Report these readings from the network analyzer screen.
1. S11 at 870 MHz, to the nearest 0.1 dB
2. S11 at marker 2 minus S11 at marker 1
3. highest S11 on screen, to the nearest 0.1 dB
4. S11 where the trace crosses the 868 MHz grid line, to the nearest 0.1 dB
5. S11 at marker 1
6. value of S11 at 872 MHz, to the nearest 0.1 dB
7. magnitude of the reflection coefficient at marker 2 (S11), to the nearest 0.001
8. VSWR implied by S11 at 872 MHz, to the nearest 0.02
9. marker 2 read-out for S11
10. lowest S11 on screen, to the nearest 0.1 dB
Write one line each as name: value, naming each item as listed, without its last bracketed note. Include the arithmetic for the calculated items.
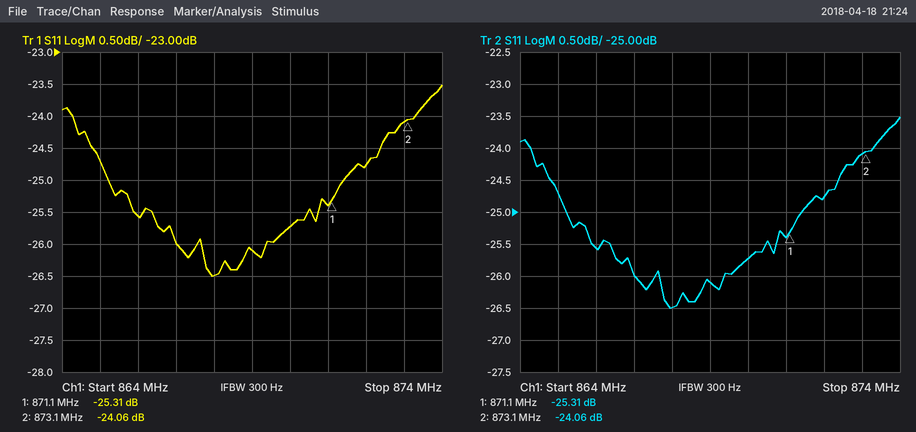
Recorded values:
S11 at 870 MHz, to the nearest 0.1 dB: -25.7 dB
S11 at marker 2 minus S11 at marker 1: -24.06 − (-25.31) = 1.25 dB
highest S11 on screen, to the nearest 0.1 dB: -23.5 dB
S11 where the trace crosses the 868 MHz grid line, to the nearest 0.1 dB: -26.5 dB
S11 at marker 1: -25.31 dB
value of S11 at 872 MHz, to the nearest 0.1 dB: -24.8 dB
magnitude of the reflection coefficient at marker 2 (S11), to the nearest 0.001: 10^(-24.06/20) ≈ 0.063
VSWR implied by S11 at 872 MHz, to the nearest 0.02: |Γ| = 10^(-24.8/20) = 0.0575; VSWR = (1 + 0.0575)/(1 − 0.0575) ≈ 1.12
marker 2 read-out for S11: -24.06 dB
lowest S11 on screen, to the nearest 0.1 dB: -26.5 dB
